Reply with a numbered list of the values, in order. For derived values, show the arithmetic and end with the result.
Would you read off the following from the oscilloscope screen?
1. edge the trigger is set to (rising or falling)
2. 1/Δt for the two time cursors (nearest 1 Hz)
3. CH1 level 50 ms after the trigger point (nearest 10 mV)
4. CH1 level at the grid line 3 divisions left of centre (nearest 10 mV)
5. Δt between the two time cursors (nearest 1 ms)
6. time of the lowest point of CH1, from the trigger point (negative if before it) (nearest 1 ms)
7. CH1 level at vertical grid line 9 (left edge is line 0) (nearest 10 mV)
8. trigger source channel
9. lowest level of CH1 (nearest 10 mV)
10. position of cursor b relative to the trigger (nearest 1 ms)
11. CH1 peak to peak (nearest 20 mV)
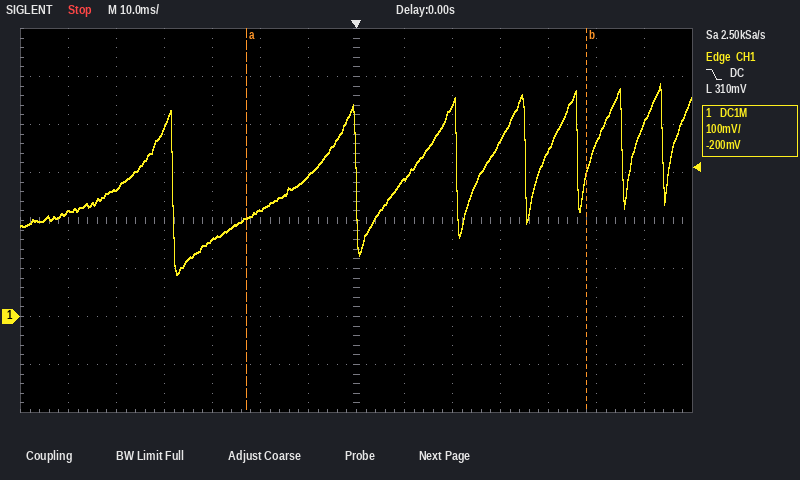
1. falling
2. 1 / 71 ms ≈ 14 Hz
3. 360 mV
4. 160 mV
5. 71 ms
6. -37 ms
7. 440 mV
8. CH1
9. 90 mV
10. +48 ms
11. 400 mV
